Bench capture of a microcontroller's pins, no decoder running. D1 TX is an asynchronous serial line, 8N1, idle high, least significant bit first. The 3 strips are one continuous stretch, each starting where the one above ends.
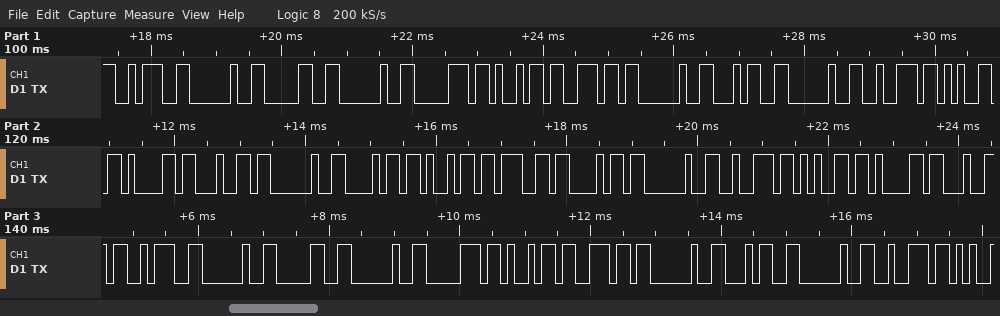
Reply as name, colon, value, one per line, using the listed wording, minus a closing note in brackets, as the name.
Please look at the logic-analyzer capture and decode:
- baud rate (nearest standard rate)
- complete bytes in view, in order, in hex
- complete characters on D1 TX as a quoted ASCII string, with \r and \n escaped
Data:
baud rate: 9600 baud
complete bytes in view, in order, in hex: 3A 20 30 20 70 69 6E 20 34 20 72 65 61 64 20 68 69 67 68 20 72 65 61 64 3A 20 30 20 70 69 6E 20 34 20 72
complete characters on D1 TX as a quoted ASCII string, with \r and \n escaped: ": 0 pin 4 read high read: 0 pin 4 r"
